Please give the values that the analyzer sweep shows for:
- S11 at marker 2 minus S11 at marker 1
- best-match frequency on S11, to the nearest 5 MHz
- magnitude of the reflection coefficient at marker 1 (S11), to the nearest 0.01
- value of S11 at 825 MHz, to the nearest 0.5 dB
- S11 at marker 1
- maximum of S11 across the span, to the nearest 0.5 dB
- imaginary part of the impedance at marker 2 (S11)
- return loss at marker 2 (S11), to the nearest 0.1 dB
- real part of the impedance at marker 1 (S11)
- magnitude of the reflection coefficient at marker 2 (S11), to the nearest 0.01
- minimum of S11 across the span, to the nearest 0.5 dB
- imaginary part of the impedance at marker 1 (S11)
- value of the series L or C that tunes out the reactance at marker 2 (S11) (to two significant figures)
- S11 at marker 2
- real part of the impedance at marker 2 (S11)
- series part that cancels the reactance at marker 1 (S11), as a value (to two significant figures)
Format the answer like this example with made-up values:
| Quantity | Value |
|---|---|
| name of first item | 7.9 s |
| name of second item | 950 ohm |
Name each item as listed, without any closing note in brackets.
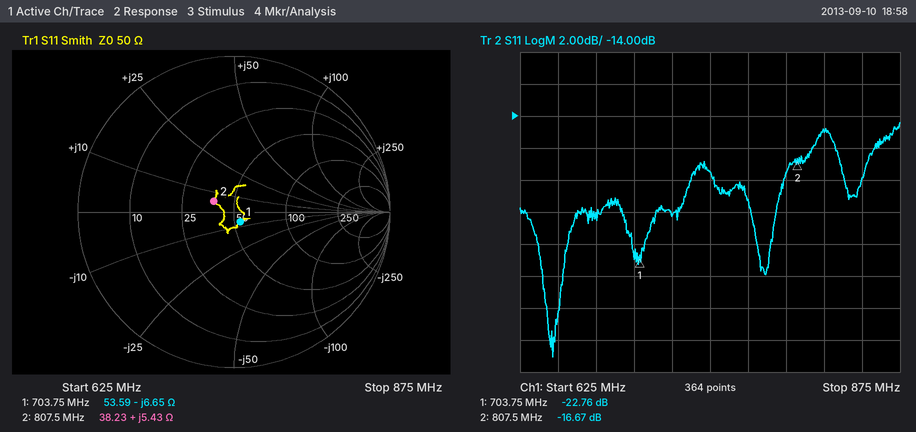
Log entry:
| Quantity | Value |
|---|---|
| S11 at marker 2 minus S11 at marker 1 | 6.09 dB |
| best-match frequency on S11, to the nearest 5 MHz | 645 MHz |
| magnitude of the reflection coefficient at marker 1 (S11), to the nearest 0.01 | 0.07 |
| value of S11 at 825 MHz, to the nearest 0.5 dB | -15.0 dB |
| S11 at marker 1 | -22.76 dB |
| maximum of S11 across the span, to the nearest 0.5 dB | -14.5 dB |
| imaginary part of the impedance at marker 2 | +5.43 Ω |
| return loss at marker 2 (S11), to the nearest 0.1 dB | 16.7 dB |
| real part of the impedance at marker 1 | 53.59 Ω |
| magnitude of the reflection coefficient at marker 2 (S11), to the nearest 0.01 | 0.15 |
| minimum of S11 across the span, to the nearest 0.5 dB | -29.0 dB |
| imaginary part of the impedance at marker 1 | -6.65 Ω |
| value of the series L or C that tunes out the reactance at marker 2 (S11) | 36 pF |
| S11 at marker 2 | -16.67 dB |
| real part of the impedance at marker 2 | 38.23 Ω |
| series part that cancels the reactance at marker 1 (S11), as a value | 1.5 nH |
